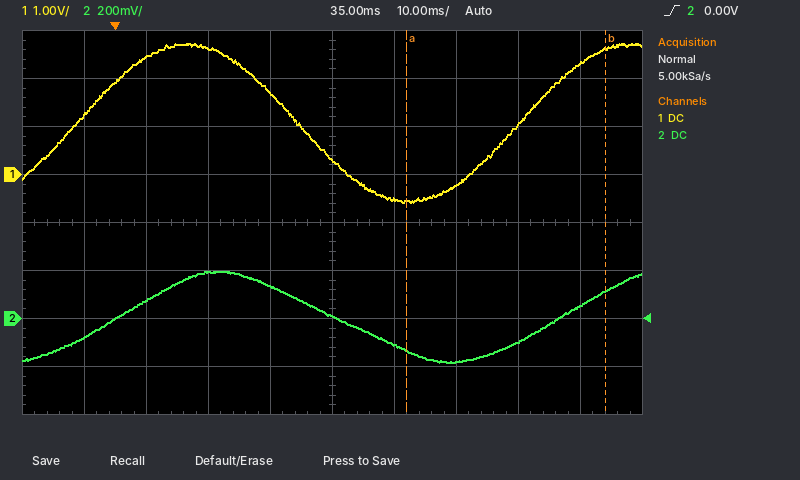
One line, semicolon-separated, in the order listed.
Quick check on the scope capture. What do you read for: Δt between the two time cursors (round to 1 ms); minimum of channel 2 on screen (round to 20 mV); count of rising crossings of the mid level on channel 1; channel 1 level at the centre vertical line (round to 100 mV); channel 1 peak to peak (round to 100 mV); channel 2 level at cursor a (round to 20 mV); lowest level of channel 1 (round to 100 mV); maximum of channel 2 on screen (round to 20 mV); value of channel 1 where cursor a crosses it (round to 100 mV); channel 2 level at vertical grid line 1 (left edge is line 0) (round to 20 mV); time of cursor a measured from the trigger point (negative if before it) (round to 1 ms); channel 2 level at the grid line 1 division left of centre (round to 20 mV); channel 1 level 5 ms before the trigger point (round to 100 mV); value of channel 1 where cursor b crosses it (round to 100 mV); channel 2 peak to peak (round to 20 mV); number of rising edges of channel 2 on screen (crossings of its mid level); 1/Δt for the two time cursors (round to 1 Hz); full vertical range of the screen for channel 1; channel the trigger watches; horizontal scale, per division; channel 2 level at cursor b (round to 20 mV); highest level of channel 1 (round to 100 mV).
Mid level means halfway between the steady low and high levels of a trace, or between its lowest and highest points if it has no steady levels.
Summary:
32 ms; -180 mV; 2; 300 mV; 3.3 V; -140 mV; -600 mV; 200 mV; -600 mV; -80 mV; +47 ms; 140 mV; 1.2 V; 2.6 V; 380 mV; 2; 31 Hz; 8 V; channel 2; 10 ms; 120 mV; 2.7 V
